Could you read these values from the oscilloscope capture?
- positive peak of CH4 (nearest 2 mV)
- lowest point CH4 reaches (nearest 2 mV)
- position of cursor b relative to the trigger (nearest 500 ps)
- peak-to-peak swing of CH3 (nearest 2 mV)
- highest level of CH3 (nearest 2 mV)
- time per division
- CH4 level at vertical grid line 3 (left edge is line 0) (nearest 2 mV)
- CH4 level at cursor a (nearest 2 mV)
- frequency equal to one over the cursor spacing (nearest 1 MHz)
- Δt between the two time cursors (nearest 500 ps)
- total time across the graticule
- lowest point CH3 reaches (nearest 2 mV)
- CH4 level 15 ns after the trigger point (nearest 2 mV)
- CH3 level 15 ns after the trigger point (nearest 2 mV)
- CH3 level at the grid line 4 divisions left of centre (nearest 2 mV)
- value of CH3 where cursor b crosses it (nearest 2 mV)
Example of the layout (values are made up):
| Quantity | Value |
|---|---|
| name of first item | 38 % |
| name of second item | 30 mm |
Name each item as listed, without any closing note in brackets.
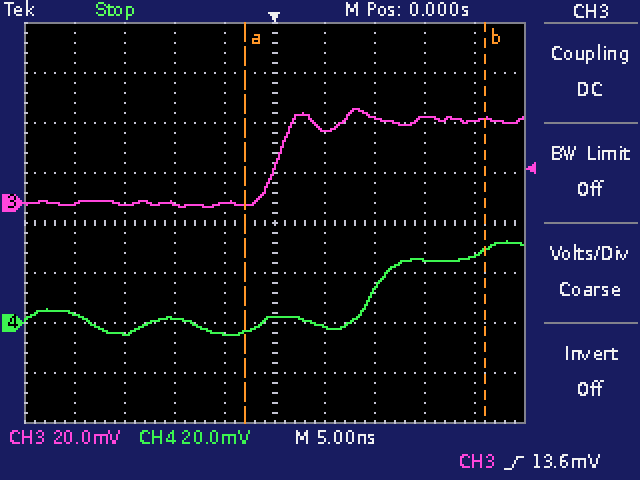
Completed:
| Quantity | Value |
|---|---|
| positive peak of CH4 | 32 mV |
| lowest point CH4 reaches | -4 mV |
| position of cursor b relative to the trigger | +21.0 ns |
| peak-to-peak swing of CH3 | 40 mV |
| highest level of CH3 | 38 mV |
| time per division | 5 ns |
| CH4 level at vertical grid line 3 (left edge is line 0) | 2 mV |
| CH4 level at cursor a | -4 mV |
| frequency equal to one over the cursor spacing | 42 MHz |
| Δt between the two time cursors | 24.0 ns |
| total time across the graticule | 50 ns |
| lowest point CH3 reaches | -2 mV |
| CH4 level 15 ns after the trigger point | 26 mV |
| CH3 level 15 ns after the trigger point | 34 mV |
| CH3 level at the grid line 4 divisions left of centre | 0 mV |
| value of CH3 where cursor b crosses it | 34 mV |
